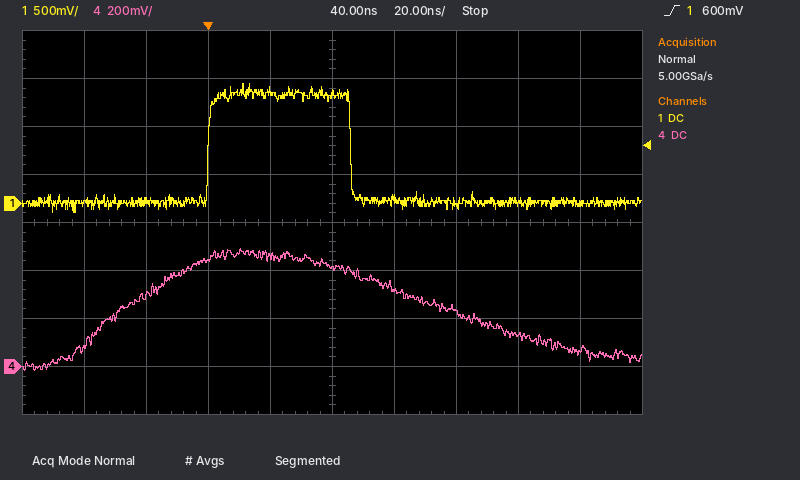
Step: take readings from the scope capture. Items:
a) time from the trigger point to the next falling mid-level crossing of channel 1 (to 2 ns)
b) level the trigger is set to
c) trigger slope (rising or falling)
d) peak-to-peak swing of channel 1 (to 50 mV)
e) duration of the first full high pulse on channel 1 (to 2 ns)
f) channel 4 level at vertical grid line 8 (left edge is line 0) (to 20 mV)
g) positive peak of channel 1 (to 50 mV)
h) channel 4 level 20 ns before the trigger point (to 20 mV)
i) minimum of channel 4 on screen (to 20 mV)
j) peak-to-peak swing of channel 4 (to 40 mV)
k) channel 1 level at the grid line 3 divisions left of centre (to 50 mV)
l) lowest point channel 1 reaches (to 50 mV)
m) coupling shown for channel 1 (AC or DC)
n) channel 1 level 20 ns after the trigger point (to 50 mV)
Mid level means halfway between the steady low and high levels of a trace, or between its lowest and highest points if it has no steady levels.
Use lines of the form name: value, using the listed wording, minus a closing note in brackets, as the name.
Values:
time from the trigger point to the next falling mid-level crossing of channel 1: 46 ns
level the trigger is set to: 600 mV
trigger slope: rising
peak-to-peak swing of channel 1: 1.35 V
duration of the first full high pulse on channel 1: 46 ns
channel 4 level at vertical grid line 8 (left edge is line 0): 140 mV
positive peak of channel 1: 1.25 V
channel 4 level 20 ns before the trigger point: 300 mV
minimum of channel 4 on screen: -20 mV
peak-to-peak swing of channel 4: 520 mV
channel 1 level at the grid line 3 divisions left of centre: 0 mV
lowest point channel 1 reaches: -100 mV
coupling shown for channel 1: DC
channel 1 level 20 ns after the trigger point: 1.15 V
